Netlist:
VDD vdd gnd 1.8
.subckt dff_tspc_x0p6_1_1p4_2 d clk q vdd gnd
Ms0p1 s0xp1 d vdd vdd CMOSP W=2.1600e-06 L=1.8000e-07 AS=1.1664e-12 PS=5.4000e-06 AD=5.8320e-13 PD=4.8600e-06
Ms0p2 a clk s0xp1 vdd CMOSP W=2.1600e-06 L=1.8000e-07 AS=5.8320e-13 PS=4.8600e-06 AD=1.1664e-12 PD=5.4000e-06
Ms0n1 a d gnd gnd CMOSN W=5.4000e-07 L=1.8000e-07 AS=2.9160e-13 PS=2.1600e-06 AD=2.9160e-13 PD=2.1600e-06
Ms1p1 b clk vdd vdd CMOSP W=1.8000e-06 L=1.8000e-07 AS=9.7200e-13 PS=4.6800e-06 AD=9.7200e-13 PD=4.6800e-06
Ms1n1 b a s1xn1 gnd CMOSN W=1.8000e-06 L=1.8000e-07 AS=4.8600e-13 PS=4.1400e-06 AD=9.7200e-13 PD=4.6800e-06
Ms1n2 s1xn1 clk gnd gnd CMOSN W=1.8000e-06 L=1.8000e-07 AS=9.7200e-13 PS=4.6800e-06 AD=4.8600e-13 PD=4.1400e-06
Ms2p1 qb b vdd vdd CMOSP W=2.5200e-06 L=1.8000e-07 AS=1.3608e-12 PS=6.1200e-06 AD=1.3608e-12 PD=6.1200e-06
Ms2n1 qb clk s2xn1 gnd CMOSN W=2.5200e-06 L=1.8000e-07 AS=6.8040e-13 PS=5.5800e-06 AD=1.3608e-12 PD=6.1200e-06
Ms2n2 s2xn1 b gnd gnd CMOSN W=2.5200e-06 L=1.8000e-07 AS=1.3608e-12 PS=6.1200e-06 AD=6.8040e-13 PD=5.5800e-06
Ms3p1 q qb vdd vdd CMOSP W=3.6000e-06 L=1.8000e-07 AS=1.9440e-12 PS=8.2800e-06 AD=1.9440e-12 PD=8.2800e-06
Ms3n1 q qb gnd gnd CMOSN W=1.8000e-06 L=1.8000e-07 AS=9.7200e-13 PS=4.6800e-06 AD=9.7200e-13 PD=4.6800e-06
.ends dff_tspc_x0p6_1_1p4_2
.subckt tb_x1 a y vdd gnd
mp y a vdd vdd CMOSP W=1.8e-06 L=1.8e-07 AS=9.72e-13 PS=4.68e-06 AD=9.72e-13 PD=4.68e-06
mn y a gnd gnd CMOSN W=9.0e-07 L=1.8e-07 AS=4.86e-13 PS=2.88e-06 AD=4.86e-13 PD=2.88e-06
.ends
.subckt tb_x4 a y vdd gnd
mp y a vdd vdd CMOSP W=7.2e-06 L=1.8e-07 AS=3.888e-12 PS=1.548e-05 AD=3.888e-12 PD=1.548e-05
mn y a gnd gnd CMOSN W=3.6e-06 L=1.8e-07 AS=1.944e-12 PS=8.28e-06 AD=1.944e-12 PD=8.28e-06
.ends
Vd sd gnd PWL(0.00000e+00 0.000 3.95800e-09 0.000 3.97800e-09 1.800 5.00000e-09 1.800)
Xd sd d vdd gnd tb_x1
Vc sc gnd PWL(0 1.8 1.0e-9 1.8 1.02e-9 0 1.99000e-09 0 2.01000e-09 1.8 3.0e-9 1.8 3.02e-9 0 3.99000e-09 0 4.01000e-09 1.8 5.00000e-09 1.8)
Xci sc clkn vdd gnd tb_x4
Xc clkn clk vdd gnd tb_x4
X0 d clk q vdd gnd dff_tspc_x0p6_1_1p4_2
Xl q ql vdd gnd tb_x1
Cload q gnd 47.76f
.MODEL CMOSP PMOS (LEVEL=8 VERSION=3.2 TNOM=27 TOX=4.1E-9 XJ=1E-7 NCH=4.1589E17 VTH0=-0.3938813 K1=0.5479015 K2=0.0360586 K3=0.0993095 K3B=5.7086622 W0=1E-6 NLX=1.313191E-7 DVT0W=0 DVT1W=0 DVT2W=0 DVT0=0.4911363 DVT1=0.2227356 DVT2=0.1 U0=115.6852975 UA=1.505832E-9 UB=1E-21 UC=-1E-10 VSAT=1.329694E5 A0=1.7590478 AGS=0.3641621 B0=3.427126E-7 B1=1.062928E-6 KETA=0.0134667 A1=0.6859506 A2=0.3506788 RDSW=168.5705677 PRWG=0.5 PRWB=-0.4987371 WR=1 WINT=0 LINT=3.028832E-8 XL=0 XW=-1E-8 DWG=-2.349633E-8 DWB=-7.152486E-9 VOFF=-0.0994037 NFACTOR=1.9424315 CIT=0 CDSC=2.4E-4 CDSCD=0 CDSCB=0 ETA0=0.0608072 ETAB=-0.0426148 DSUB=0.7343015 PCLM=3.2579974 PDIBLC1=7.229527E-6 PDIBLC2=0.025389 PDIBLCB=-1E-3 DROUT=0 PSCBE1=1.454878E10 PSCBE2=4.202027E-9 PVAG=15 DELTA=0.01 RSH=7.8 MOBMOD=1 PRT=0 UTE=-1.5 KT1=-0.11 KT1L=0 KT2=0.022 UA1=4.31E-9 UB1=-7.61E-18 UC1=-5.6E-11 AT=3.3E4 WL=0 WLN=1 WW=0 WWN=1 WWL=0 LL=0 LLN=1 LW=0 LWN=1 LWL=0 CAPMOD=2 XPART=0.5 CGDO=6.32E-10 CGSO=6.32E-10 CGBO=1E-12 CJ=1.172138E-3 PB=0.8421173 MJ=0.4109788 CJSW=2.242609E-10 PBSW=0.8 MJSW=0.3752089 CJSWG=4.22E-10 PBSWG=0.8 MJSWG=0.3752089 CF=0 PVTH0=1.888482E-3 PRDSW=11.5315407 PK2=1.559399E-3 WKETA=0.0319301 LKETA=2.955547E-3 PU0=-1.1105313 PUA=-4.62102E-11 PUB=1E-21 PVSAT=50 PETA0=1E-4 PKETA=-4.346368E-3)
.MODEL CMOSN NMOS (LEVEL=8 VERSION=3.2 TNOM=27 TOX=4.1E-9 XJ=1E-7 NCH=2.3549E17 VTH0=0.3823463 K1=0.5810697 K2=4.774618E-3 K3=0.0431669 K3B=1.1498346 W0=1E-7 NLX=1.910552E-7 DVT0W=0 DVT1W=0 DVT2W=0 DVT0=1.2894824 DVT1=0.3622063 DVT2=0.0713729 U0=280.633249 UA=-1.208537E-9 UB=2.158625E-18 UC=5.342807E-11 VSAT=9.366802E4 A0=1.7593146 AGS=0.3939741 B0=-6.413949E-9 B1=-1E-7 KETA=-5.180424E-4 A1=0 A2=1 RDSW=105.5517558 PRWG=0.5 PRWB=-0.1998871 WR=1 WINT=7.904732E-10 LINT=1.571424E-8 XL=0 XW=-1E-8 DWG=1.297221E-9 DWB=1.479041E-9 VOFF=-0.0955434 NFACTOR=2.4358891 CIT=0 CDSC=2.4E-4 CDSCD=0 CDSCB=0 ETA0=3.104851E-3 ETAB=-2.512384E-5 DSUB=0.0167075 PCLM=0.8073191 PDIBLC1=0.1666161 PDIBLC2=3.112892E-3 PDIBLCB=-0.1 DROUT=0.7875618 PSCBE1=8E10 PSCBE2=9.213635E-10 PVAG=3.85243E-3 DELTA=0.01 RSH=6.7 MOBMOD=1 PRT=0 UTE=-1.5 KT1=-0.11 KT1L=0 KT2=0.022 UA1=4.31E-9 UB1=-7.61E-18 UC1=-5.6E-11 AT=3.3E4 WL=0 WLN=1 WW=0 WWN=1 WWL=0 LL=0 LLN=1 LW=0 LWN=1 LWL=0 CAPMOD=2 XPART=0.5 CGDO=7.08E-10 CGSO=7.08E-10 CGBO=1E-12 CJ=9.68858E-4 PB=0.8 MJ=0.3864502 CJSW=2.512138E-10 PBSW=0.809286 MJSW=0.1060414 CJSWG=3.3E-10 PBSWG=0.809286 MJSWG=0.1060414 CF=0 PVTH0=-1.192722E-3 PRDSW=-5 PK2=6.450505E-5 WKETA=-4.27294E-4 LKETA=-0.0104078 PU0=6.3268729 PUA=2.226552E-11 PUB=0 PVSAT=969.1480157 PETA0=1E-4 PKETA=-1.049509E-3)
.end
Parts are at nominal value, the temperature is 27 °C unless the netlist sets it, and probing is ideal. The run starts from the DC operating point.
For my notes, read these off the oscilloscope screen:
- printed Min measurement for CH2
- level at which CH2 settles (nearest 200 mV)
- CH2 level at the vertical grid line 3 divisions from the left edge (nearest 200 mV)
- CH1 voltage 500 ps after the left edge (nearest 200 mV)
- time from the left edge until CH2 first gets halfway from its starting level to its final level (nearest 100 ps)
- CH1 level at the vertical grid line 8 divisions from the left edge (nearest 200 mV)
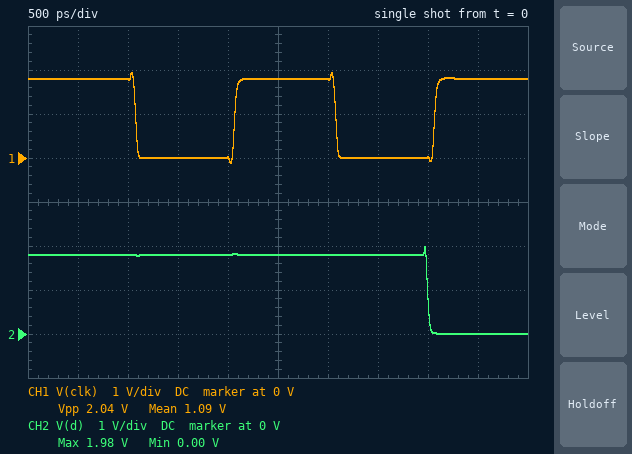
0.00 V
0 V
1.8 V
1.8 V
4.0 ns
0 V
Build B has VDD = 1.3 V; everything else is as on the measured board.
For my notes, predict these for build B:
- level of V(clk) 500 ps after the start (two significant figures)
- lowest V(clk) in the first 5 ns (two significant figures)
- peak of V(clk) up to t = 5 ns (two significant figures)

1.3 V
-170 mV
1.4 V
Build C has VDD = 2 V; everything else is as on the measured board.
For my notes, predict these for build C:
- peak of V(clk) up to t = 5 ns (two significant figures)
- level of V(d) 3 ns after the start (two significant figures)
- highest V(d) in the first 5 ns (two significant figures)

2.1 V
2.0 V
2.2 V
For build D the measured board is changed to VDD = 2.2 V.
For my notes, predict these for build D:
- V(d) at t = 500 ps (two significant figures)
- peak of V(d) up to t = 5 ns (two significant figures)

2.2 V
2.4 V
